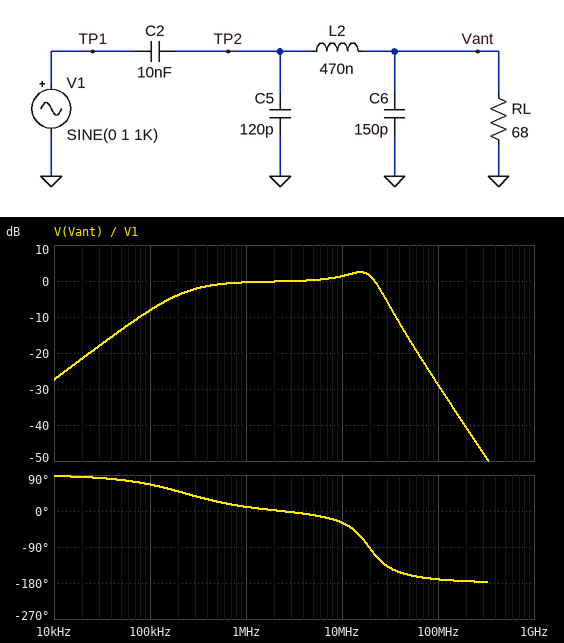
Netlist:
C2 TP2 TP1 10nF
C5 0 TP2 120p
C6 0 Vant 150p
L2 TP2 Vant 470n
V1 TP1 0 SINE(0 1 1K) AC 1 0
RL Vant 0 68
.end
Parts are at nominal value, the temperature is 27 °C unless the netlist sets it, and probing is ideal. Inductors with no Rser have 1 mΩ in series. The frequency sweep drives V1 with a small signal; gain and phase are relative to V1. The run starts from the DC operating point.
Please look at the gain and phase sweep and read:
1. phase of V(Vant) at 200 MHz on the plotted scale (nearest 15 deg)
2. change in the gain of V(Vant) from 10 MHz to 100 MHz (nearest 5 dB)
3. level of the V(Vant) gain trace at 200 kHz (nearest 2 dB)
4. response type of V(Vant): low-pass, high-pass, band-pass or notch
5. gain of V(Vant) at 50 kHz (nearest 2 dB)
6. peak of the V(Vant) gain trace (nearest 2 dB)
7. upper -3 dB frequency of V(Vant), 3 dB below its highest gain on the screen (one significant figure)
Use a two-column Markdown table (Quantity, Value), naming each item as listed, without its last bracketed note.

| Quantity | Value |
|---|---|
| phase of V(Vant) at 200 MHz on the plotted scale | -180 deg |
| change in the gain of V(Vant) from 10 MHz to 100 MHz | -30 dB |
| level of the V(Vant) gain trace at 200 kHz | -4 dB |
| response type of V(Vant): low-pass, high-pass, band-pass or notch | band-pass |
| gain of V(Vant) at 50 kHz | -14 dB |
| peak of the V(Vant) gain trace | 2 dB |
| upper -3 dB frequency of V(Vant), 3 dB below its highest gain on the screen | 20 MHz |
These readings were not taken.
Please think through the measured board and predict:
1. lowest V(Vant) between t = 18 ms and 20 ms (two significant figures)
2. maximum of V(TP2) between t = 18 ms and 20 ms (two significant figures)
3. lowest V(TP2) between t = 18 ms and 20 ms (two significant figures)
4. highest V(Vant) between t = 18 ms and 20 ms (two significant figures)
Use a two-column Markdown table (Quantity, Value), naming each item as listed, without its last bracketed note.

| Quantity | Value |
|---|---|
| lowest V(Vant) between t = 18 ms and 20 ms | -4.3 mV |
| maximum of V(TP2) between t = 18 ms and 20 ms | 4.3 mV |
| lowest V(TP2) between t = 18 ms and 20 ms | -4.3 mV |
| highest V(Vant) between t = 18 ms and 20 ms | 4.3 mV |
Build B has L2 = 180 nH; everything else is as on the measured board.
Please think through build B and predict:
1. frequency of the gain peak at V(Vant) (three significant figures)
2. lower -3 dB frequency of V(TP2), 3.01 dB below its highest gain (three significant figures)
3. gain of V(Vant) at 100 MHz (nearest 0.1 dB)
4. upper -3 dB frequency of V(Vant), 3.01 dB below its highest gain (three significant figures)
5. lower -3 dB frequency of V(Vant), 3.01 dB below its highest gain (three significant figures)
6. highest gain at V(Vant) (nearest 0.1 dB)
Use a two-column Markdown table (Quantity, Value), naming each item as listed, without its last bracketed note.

| Quantity | Value |
|---|---|
| frequency of the gain peak at V(Vant) | 28.8 MHz |
| lower -3 dB frequency of V(TP2), 3.01 dB below its highest gain | 244 kHz |
| gain of V(Vant) at 100 MHz | -19.9 dB |
| upper -3 dB frequency of V(Vant), 3.01 dB below its highest gain | 35.9 MHz |
| lower -3 dB frequency of V(Vant), 3.01 dB below its highest gain | 19.3 MHz |
| highest gain at V(Vant) | 6.1 dB |
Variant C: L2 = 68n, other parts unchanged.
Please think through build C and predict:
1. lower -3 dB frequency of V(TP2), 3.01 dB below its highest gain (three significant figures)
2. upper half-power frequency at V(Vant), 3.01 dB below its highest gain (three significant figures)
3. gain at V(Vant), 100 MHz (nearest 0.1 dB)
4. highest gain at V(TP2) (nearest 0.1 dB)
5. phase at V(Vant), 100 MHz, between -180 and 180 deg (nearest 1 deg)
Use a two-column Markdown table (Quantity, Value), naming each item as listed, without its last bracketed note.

| Quantity | Value |
|---|---|
| lower -3 dB frequency of V(TP2), 3.01 dB below its highest gain | 249 kHz |
| upper half-power frequency at V(Vant), 3.01 dB below its highest gain | 56.2 MHz |
| gain at V(Vant), 100 MHz | -9.9 dB |
| highest gain at V(TP2) | 0.1 dB |
| phase at V(Vant), 100 MHz, between -180 and 180 deg | -168 deg |
